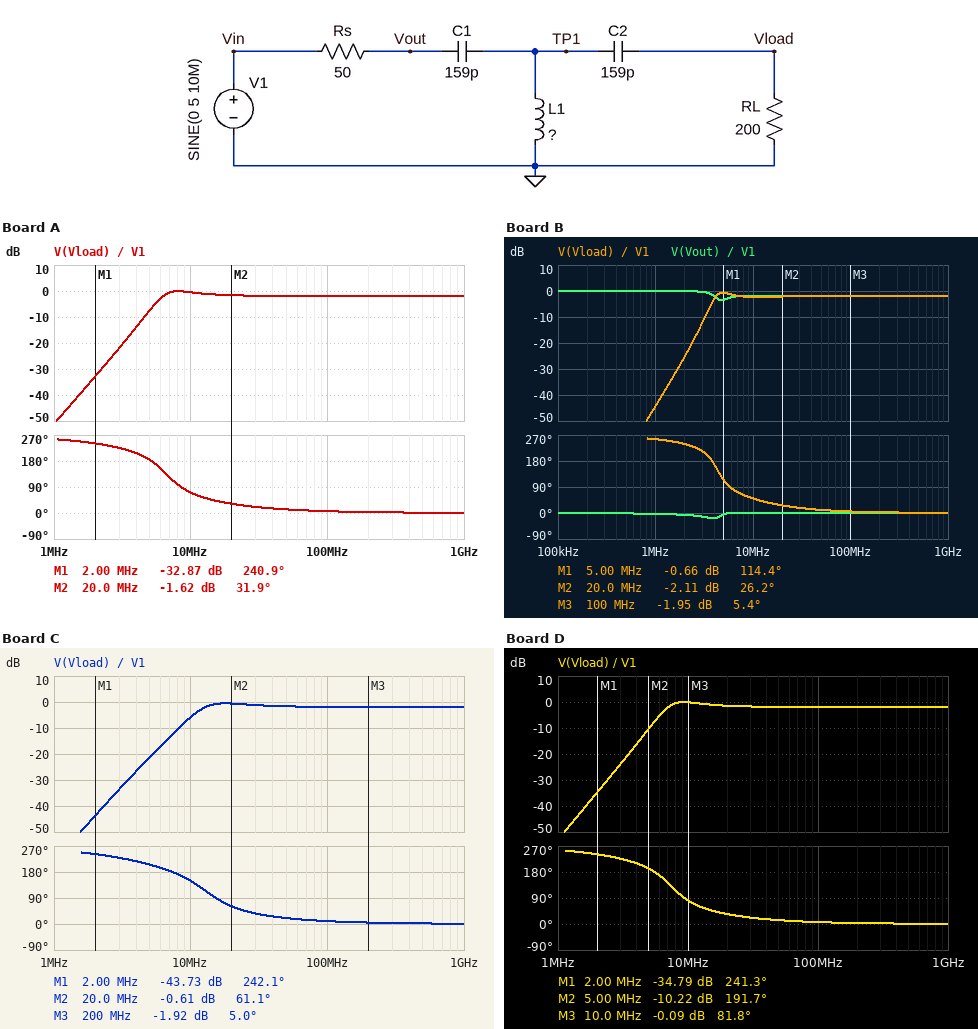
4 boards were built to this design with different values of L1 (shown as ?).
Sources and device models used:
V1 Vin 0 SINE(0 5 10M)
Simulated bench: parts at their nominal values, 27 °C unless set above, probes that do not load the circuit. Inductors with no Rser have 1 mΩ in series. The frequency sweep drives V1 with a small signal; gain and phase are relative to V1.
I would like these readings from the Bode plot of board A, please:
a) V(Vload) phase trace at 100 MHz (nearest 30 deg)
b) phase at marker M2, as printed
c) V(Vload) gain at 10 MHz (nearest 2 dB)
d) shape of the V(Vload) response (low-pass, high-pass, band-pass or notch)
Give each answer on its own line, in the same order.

0 deg
31.9 deg
0 dB
high-pass
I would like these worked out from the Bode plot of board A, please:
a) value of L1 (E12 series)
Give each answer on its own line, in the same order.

2.2 µH
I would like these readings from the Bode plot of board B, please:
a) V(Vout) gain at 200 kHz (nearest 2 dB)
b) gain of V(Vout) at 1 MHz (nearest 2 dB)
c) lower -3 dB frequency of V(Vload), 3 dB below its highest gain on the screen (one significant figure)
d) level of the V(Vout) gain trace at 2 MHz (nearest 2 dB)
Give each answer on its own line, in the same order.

0 dB
0 dB
4 MHz
0 dB
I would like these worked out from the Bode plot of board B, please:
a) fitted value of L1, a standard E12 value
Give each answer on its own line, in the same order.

4.7 µH
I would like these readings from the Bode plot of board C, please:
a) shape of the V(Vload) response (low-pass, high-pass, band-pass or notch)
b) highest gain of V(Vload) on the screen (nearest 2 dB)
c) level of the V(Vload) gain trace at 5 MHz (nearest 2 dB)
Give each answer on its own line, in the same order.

high-pass
0 dB
-22 dB
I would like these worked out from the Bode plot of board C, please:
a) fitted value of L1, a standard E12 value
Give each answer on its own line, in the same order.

680 nH
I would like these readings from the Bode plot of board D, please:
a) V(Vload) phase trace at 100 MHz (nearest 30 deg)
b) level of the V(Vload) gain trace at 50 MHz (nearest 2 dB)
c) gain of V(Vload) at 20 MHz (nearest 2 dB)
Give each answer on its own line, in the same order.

0 deg
-2 dB
-2 dB
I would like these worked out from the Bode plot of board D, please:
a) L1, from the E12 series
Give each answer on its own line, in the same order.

1.8 µH
